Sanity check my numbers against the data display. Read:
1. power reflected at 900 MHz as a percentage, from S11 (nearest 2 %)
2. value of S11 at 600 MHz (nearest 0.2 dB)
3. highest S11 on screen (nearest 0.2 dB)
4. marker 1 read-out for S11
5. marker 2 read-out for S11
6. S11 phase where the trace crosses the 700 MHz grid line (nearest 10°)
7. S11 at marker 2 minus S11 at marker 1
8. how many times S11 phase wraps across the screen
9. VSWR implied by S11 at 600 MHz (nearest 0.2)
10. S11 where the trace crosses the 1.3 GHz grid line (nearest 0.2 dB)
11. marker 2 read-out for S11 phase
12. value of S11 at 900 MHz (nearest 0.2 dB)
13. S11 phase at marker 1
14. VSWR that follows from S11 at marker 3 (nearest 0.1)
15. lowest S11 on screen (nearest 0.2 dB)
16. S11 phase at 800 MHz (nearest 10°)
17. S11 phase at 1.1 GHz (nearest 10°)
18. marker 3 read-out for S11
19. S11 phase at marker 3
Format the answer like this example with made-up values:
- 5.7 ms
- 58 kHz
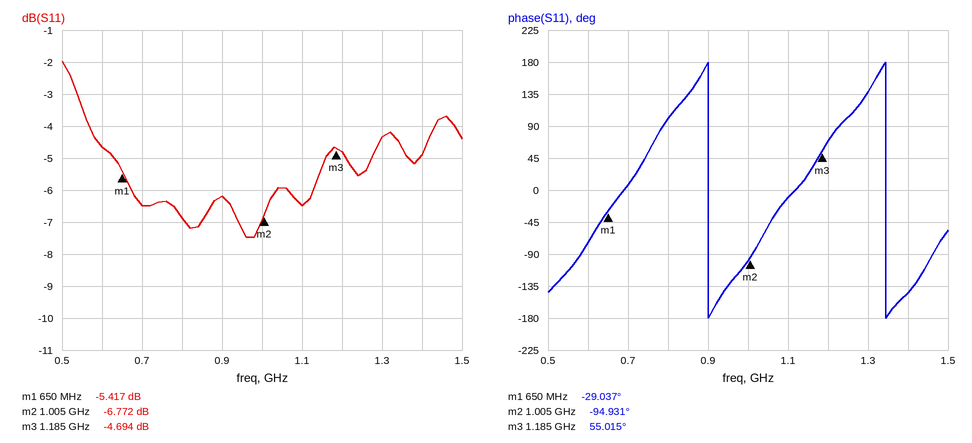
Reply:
- 24 %
- -4.6 dB
- -2.0 dB
- -5.417 dB
- -6.772 dB
- 10°
- -1.355 dB
- 2
- 3.8
- -4.4 dB
- -94.931°
- -6.2 dB
- -29.037°
- 3.8
- -7.4 dB
- 100°
- -10°
- -4.694 dB
- 55.015°
